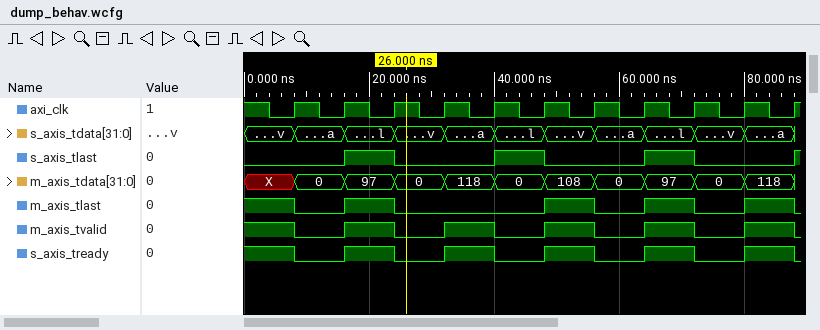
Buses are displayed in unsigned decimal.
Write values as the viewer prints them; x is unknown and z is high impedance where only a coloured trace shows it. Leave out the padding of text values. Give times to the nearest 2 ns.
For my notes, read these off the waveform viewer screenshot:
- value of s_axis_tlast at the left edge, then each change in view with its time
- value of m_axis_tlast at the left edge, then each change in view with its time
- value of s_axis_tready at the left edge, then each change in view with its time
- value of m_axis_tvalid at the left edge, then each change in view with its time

0, 1 at 16 ns, 0 at 24 ns, 1 at 40 ns, 0 at 48 ns, 1 at 64 ns, 0 at 72 ns, 1 at 88 ns
1, 0 at 8 ns, 1 at 16 ns, 0 at 24 ns, 1 at 48 ns, 0 at 56 ns, 1 at 64 ns, 0 at 72 ns, 1 at 80 ns, 0 at 88 ns
1, 0 at 8 ns, 1 at 16 ns, 0 at 24 ns, 1 at 32 ns, 0 at 40 ns, 1 at 48 ns, 0 at 56 ns, 1 at 64 ns, 0 at 72 ns, 1 at 80 ns, 0 at 88 ns
1, 0 at 8 ns, 1 at 16 ns, 0 at 24 ns, 1 at 32 ns, 0 at 40 ns, 1 at 48 ns, 0 at 56 ns, 1 at 64 ns, 0 at 72 ns, 1 at 80 ns, 0 at 88 ns
